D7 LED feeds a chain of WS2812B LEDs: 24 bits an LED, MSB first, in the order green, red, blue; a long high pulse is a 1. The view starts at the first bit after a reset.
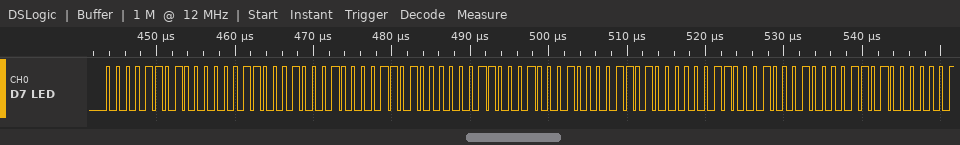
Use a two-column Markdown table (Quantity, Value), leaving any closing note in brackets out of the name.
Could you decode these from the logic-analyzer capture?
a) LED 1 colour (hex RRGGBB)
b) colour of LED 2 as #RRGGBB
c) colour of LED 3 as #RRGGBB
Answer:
| Quantity | Value |
|---|---|
| LED 1 colour | #030D11 |
| colour of LED 2 as #RRGGBB | #030D11 |
| colour of LED 3 as #RRGGBB | #030D11 |
